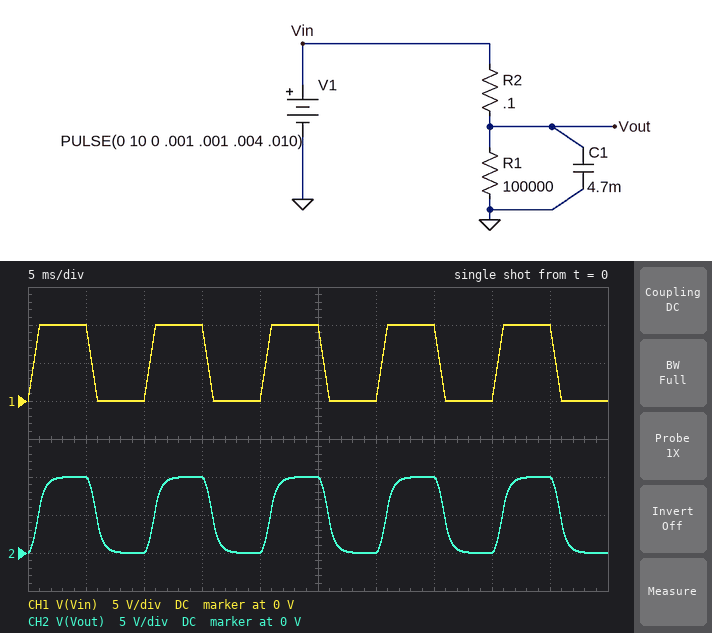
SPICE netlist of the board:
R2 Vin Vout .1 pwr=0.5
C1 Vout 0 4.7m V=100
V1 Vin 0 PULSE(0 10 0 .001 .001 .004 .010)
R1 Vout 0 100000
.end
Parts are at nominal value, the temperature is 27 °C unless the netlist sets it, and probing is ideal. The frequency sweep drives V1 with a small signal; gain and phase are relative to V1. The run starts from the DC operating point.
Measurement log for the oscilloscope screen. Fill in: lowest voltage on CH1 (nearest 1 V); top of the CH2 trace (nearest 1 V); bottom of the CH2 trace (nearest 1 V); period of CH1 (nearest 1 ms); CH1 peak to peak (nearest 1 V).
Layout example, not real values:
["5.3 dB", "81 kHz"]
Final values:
["0 V", "10 V", "0 V", "10 ms", "10 V"]
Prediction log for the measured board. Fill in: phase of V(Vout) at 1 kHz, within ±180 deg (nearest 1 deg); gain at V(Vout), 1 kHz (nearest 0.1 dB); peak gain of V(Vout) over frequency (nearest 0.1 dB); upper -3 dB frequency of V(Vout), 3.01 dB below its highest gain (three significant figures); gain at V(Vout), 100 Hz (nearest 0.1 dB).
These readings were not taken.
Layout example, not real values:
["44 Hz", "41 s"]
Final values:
["-71 deg", "-9.9 dB", "0 dB", "339 Hz", "-0.4 dB"]
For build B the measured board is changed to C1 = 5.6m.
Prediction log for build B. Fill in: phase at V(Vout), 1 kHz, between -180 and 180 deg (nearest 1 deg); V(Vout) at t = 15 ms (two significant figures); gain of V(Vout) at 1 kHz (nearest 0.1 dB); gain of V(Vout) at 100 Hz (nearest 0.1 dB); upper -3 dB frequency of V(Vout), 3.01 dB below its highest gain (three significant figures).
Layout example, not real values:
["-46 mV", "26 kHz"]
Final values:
["-74 deg", "10 V", "-11.3 dB", "-0.5 dB", "284 Hz"]
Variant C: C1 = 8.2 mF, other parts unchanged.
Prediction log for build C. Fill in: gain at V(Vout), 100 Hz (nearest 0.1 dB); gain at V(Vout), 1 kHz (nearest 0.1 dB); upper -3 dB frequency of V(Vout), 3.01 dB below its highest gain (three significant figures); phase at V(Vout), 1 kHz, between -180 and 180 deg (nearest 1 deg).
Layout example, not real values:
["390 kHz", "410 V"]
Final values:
["-1.0 dB", "-14.4 dB", "194 Hz", "-79 deg"]
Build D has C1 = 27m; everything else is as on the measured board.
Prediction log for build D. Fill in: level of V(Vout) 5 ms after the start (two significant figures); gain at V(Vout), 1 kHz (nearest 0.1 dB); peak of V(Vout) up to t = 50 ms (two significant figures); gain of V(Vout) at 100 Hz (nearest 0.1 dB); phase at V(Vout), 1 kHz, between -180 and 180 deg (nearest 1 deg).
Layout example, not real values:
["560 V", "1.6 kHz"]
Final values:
["8.1 V", "-24.6 dB", "8.4 V", "-5.9 dB", "-87 deg"]
